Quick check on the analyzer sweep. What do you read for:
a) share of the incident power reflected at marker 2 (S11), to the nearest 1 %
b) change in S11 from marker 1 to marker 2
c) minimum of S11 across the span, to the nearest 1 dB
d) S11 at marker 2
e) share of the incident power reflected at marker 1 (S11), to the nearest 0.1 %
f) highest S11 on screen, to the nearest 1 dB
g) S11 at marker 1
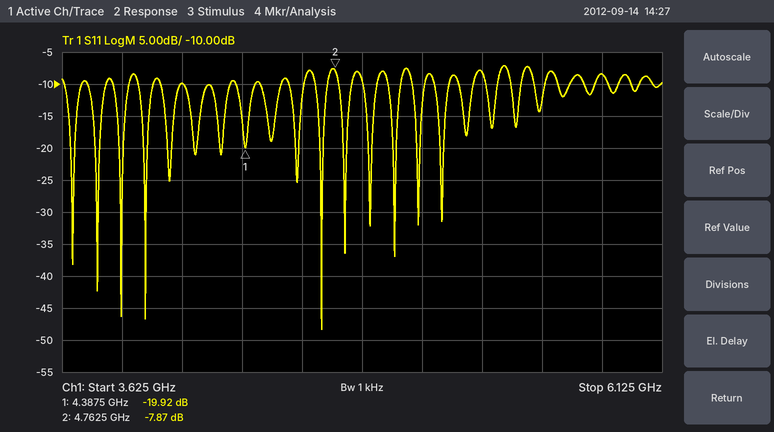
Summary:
16 %
12.05 dB
-48 dB
-7.87 dB
1.0 %
-7 dB
-19.92 dB
